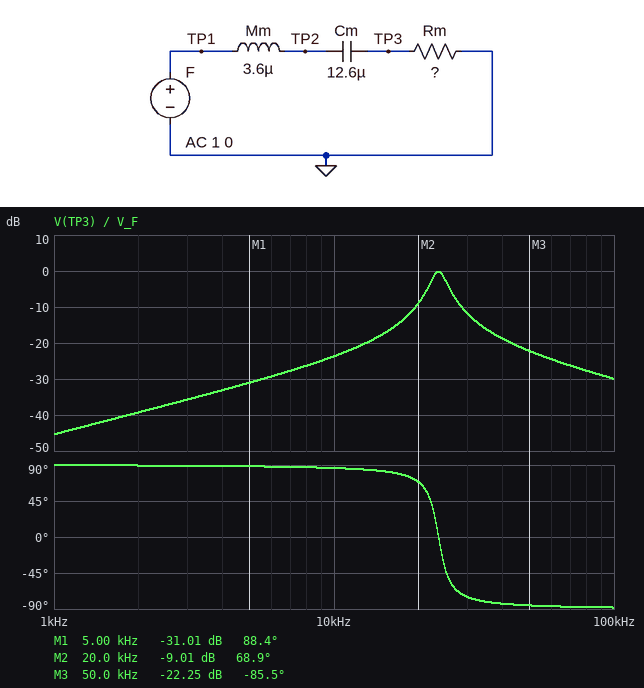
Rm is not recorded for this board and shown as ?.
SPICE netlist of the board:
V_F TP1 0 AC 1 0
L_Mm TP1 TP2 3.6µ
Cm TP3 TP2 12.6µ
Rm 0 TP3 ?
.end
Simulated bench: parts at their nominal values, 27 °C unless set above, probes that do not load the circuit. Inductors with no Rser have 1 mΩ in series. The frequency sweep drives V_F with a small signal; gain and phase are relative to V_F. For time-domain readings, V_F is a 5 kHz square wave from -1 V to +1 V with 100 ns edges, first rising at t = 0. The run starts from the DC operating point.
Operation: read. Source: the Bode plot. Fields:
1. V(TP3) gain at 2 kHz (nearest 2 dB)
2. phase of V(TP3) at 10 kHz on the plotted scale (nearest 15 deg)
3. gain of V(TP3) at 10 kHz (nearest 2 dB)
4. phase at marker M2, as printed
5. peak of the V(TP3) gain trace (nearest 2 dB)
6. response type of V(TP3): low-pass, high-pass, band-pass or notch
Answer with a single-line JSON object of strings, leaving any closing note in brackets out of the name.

{"V(TP3) gain at 2 kHz": "-40 dB", "phase of V(TP3) at 10 kHz on the plotted scale": "90 deg", "gain of V(TP3) at 10 kHz": "-24 dB", "phase at marker M2, as printed": "68.9 deg", "peak of the V(TP3) gain trace": "0 dB", "response type of V(TP3): low-pass, high-pass, band-pass or notch": "band-pass"}
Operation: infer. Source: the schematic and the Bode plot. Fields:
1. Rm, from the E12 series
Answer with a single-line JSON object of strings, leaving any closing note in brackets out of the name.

{"Rm, from the E12 series": "0.068 Ω"}
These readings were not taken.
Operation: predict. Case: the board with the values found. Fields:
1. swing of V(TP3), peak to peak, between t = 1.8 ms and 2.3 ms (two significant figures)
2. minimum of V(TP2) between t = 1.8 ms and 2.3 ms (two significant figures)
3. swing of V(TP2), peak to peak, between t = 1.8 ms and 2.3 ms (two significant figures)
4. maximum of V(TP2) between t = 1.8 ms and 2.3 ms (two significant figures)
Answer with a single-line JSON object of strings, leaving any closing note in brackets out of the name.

{"swing of V(TP3), peak to peak, between t = 1.8 ms and 2.3 ms": "550 mV", "minimum of V(TP2) between t = 1.8 ms and 2.3 ms": "-3.0 V", "swing of V(TP2), peak to peak, between t = 1.8 ms and 2.3 ms": "5.9 V", "maximum of V(TP2) between t = 1.8 ms and 2.3 ms": "3.0 V"}
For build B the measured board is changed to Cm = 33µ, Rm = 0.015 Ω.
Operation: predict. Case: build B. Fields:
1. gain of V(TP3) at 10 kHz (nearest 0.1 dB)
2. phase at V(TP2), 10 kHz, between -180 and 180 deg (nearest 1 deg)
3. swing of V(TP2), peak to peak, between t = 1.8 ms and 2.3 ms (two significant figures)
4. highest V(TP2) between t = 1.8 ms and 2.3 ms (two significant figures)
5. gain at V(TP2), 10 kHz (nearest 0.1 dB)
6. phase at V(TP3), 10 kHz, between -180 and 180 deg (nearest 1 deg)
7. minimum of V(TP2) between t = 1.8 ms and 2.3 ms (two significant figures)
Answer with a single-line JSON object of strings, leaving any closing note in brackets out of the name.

{"gain of V(TP3) at 10 kHz": "-24.7 dB", "phase at V(TP2), 10 kHz, between -180 and 180 deg": "-2 deg", "swing of V(TP2), peak to peak, between t = 1.8 ms and 2.3 ms": "14 V", "highest V(TP2) between t = 1.8 ms and 2.3 ms": "7.0 V", "gain at V(TP2), 10 kHz": "5.5 dB", "phase at V(TP3), 10 kHz, between -180 and 180 deg": "86 deg", "minimum of V(TP2) between t = 1.8 ms and 2.3 ms": "-7.0 V"}
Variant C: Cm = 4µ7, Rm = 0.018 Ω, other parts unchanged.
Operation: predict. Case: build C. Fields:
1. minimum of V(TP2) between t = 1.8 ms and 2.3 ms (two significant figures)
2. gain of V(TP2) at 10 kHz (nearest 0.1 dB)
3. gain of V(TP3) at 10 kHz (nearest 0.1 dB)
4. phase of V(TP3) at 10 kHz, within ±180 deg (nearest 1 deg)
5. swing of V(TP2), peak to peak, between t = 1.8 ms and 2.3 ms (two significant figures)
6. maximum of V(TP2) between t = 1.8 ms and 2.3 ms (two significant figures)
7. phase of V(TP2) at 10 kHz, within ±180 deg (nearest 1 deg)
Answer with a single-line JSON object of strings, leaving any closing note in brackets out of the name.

{"minimum of V(TP2) between t = 1.8 ms and 2.3 ms": "-2.2 V", "gain of V(TP2) at 10 kHz": "0.6 dB", "gain of V(TP3) at 10 kHz": "-44.9 dB", "phase of V(TP3) at 10 kHz, within ±180 deg": "90 deg", "swing of V(TP2), peak to peak, between t = 1.8 ms and 2.3 ms": "4.4 V", "maximum of V(TP2) between t = 1.8 ms and 2.3 ms": "2.2 V", "phase of V(TP2) at 10 kHz, within ±180 deg": "0 deg"}
